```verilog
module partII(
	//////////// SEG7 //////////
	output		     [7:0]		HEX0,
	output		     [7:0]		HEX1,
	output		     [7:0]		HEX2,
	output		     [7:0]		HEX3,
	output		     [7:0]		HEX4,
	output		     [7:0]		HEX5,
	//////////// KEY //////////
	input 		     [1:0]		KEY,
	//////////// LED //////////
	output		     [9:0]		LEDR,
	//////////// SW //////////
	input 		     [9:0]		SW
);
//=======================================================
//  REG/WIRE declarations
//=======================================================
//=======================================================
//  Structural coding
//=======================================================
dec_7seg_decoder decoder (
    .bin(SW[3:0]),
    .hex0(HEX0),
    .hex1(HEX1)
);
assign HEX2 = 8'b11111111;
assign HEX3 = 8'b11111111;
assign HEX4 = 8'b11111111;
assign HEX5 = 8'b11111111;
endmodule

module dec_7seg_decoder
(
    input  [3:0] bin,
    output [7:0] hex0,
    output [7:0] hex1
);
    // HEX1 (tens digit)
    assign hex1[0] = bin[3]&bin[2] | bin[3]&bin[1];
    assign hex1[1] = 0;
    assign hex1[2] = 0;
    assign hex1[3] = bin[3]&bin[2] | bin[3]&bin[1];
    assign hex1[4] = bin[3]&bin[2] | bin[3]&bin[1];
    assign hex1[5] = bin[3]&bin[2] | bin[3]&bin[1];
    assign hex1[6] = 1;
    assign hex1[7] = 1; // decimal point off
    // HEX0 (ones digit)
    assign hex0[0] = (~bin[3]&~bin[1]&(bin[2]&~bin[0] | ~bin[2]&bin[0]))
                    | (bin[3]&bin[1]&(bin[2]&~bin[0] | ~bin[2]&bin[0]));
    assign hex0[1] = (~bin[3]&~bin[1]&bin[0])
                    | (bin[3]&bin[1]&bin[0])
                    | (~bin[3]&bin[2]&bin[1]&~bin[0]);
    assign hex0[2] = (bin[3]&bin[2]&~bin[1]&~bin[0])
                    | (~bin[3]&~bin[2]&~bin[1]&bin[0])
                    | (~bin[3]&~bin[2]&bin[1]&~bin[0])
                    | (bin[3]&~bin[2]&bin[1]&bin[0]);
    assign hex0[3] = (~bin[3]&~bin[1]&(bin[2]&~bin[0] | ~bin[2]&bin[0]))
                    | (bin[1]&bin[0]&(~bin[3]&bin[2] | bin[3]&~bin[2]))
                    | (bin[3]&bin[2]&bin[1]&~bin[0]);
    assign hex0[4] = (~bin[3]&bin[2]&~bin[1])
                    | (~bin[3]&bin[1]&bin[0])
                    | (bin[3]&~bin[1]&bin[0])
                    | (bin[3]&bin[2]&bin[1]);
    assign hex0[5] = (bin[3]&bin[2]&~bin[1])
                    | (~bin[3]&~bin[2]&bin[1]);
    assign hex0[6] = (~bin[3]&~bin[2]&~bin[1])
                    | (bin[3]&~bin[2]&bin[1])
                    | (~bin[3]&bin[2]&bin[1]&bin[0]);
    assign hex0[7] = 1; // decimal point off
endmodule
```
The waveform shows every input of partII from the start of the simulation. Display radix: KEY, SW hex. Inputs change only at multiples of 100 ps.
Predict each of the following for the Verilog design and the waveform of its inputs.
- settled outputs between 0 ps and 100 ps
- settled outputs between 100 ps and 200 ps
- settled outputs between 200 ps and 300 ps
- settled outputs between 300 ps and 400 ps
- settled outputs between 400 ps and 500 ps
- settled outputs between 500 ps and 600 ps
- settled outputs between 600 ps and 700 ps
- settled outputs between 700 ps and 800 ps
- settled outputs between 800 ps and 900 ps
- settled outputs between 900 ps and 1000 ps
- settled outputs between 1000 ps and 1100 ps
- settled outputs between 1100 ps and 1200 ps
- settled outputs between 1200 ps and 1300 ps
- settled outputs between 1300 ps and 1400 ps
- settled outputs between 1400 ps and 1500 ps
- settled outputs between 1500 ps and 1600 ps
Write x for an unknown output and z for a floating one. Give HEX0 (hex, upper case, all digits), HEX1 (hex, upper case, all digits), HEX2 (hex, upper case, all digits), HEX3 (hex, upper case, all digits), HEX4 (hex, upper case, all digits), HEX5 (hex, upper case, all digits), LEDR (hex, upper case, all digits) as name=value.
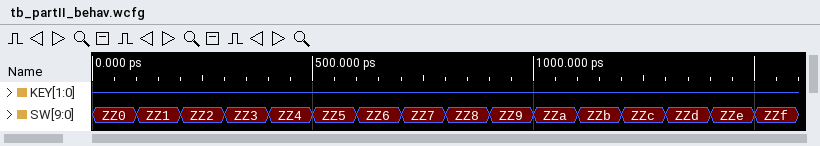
HEX0=C0, HEX1=C0, HEX2=FF, HEX3=FF, HEX4=FF, HEX5=FF, LEDR=z
HEX0=CF, HEX1=C0, HEX2=FF, HEX3=FF, HEX4=FF, HEX5=FF, LEDR=z
HEX0=A4, HEX1=C0, HEX2=FF, HEX3=FF, HEX4=FF, HEX5=FF, LEDR=z
HEX0=B0, HEX1=C0, HEX2=FF, HEX3=FF, HEX4=FF, HEX5=FF, LEDR=z
HEX0=99, HEX1=C0, HEX2=FF, HEX3=FF, HEX4=FF, HEX5=FF, LEDR=z
HEX0=92, HEX1=C0, HEX2=FF, HEX3=FF, HEX4=FF, HEX5=FF, LEDR=z
HEX0=82, HEX1=C0, HEX2=FF, HEX3=FF, HEX4=FF, HEX5=FF, LEDR=z
HEX0=D8, HEX1=C0, HEX2=FF, HEX3=FF, HEX4=FF, HEX5=FF, LEDR=z
HEX0=80, HEX1=C0, HEX2=FF, HEX3=FF, HEX4=FF, HEX5=FF, LEDR=z
HEX0=90, HEX1=C0, HEX2=FF, HEX3=FF, HEX4=FF, HEX5=FF, LEDR=z
HEX0=C0, HEX1=F9, HEX2=FF, HEX3=FF, HEX4=FF, HEX5=FF, LEDR=z
HEX0=CF, HEX1=F9, HEX2=FF, HEX3=FF, HEX4=FF, HEX5=FF, LEDR=z
HEX0=A4, HEX1=F9, HEX2=FF, HEX3=FF, HEX4=FF, HEX5=FF, LEDR=z
HEX0=B0, HEX1=F9, HEX2=FF, HEX3=FF, HEX4=FF, HEX5=FF, LEDR=z
HEX0=99, HEX1=F9, HEX2=FF, HEX3=FF, HEX4=FF, HEX5=FF, LEDR=z
HEX0=92, HEX1=F9, HEX2=FF, HEX3=FF, HEX4=FF, HEX5=FF, LEDR=z
